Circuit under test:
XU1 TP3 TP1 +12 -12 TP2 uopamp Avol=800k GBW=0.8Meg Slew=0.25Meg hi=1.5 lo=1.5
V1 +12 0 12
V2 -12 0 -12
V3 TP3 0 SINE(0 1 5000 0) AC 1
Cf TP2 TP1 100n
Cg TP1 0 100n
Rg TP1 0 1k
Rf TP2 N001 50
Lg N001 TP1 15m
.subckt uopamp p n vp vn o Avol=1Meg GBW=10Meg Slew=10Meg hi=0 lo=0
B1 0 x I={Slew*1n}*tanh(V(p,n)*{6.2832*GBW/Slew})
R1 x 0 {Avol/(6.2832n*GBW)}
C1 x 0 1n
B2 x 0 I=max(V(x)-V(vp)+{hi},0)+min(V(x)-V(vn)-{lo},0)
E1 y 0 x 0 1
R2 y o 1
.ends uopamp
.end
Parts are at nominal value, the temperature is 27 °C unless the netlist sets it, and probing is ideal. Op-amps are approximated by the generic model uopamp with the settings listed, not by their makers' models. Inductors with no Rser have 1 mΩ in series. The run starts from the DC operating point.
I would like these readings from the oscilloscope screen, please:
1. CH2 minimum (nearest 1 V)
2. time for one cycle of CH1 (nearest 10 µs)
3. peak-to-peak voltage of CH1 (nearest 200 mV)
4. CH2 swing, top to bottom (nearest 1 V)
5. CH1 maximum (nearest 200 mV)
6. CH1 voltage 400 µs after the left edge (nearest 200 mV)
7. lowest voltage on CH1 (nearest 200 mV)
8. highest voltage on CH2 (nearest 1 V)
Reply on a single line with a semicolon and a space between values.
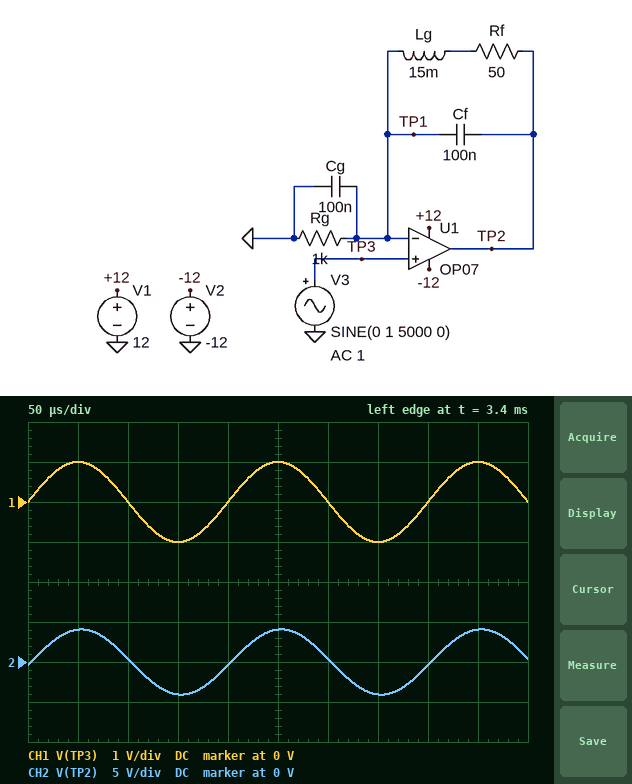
-4 V; 200 µs; 2.0 V; 8 V; 1.0 V; 0 V; -1.0 V; 4 V
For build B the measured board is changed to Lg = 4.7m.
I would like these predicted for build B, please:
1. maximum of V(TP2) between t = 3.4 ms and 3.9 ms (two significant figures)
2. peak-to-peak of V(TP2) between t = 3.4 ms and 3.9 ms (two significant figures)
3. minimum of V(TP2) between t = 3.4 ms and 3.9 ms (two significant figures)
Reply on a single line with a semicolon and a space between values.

860 mV; 1.7 V; -860 mV
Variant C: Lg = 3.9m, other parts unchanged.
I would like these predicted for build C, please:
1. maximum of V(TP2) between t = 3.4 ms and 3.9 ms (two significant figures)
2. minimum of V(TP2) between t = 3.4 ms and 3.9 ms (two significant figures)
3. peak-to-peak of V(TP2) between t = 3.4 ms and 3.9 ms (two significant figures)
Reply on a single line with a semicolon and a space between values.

820 mV; -820 mV; 1.6 V
